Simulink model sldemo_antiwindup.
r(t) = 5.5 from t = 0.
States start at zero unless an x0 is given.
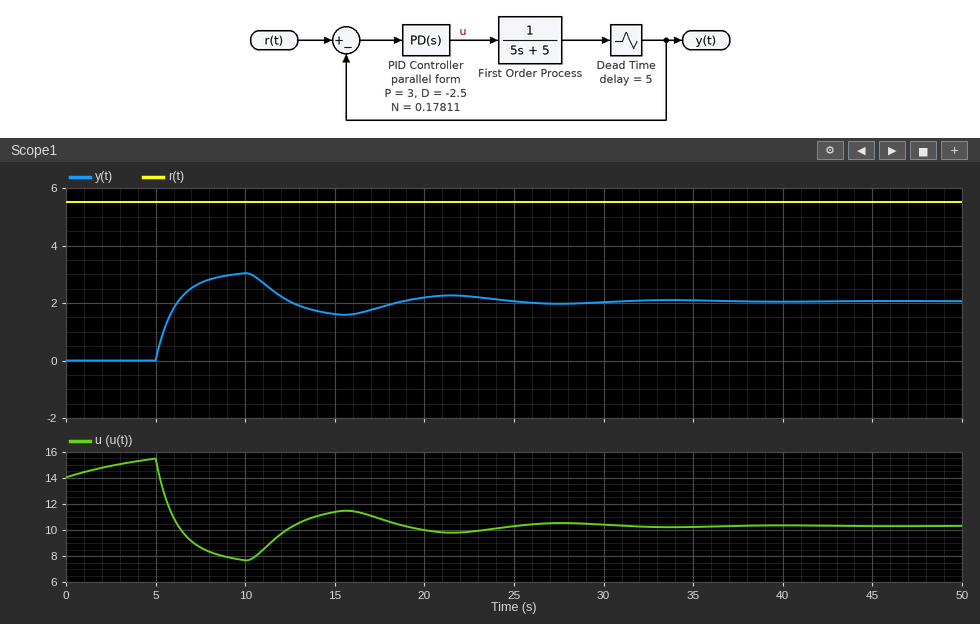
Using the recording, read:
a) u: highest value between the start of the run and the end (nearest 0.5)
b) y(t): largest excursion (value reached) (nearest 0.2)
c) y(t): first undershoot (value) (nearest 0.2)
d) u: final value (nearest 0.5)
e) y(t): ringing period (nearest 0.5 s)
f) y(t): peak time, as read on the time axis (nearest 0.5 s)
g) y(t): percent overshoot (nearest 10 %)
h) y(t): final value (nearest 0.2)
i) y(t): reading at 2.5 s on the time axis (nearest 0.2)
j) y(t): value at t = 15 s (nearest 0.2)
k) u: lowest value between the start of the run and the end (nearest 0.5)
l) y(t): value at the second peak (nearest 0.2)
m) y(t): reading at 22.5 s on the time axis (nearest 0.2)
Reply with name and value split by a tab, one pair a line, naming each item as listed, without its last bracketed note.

u: highest value between the start of the run and the end	15.5
y(t): largest excursion (value reached)	3.0
y(t): first undershoot (value)	1.6
u: final value	10.5
y(t): ringing period	11.5 s
y(t): peak time, as read on the time axis	10.0 s
y(t): percent overshoot	50 %
y(t): final value	2.0
y(t): reading at 2.5 s on the time axis	0.0
y(t): value at t = 15 s	1.6
u: lowest value between the start of the run and the end	7.5
y(t): value at the second peak	2.2
y(t): reading at 22.5 s on the time axis	2.2
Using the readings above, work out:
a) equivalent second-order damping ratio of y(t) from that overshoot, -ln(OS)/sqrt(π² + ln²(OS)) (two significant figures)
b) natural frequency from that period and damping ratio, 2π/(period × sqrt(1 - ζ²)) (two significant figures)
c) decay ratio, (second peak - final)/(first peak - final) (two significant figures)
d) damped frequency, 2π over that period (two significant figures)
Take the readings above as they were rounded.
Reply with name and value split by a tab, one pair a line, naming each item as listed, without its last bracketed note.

equivalent second-order damping ratio of y(t) from that overshoot, -ln(OS)/sqrt(π² + ln²(OS))	0.22
natural frequency from that period and damping ratio, 2π/(period × sqrt(1 - ζ²))	0.56 rad/s
decay ratio, (second peak - final)/(first peak - final)	0.20
damped frequency, 2π over that period	0.55 rad/s
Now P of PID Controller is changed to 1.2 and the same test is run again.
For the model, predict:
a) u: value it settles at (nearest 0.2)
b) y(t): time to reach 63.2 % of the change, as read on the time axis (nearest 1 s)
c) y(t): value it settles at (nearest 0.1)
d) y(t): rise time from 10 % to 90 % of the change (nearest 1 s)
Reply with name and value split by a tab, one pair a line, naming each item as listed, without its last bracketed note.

u: value it settles at	5.4
y(t): time to reach 63.2 % of the change, as read on the time axis	6 s
y(t): value it settles at	1.1
y(t): rise time from 10 % to 90 % of the change	3 s
